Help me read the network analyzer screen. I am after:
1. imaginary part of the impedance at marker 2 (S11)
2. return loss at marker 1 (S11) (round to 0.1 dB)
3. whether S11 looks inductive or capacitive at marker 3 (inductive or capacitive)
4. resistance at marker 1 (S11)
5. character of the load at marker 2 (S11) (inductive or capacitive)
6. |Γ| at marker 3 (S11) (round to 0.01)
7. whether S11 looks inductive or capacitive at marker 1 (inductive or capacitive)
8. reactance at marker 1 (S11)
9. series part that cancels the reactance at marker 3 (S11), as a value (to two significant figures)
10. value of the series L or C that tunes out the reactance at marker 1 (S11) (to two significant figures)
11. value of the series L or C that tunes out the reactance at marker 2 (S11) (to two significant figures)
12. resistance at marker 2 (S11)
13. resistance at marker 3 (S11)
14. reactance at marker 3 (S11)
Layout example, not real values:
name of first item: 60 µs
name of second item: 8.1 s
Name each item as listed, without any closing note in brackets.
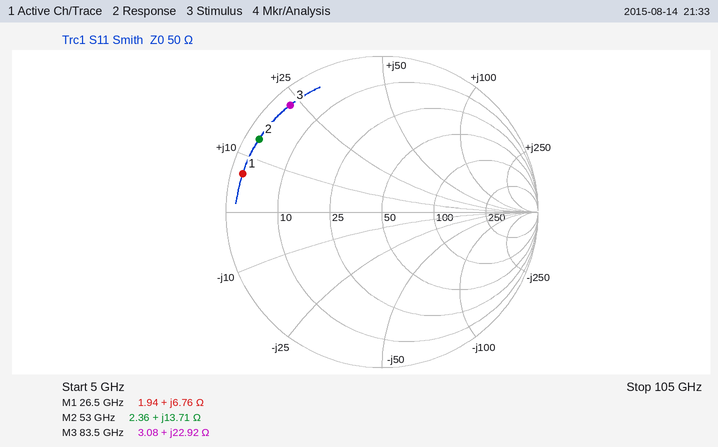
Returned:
imaginary part of the impedance at marker 2: +13.71 Ω
return loss at marker 1 (S11): 0.7 dB
whether S11 looks inductive or capacitive at marker 3: inductive
resistance at marker 1: 1.94 Ω
character of the load at marker 2 (S11): inductive
|Γ| at marker 3 (S11): 0.90
whether S11 looks inductive or capacitive at marker 1: inductive
reactance at marker 1: +6.76 Ω
series part that cancels the reactance at marker 3 (S11), as a value: 83 fF
value of the series L or C that tunes out the reactance at marker 1 (S11): 890 fF
value of the series L or C that tunes out the reactance at marker 2 (S11): 220 fF
resistance at marker 2: 2.36 Ω
resistance at marker 3: 3.08 Ω
reactance at marker 3: +22.92 Ω
